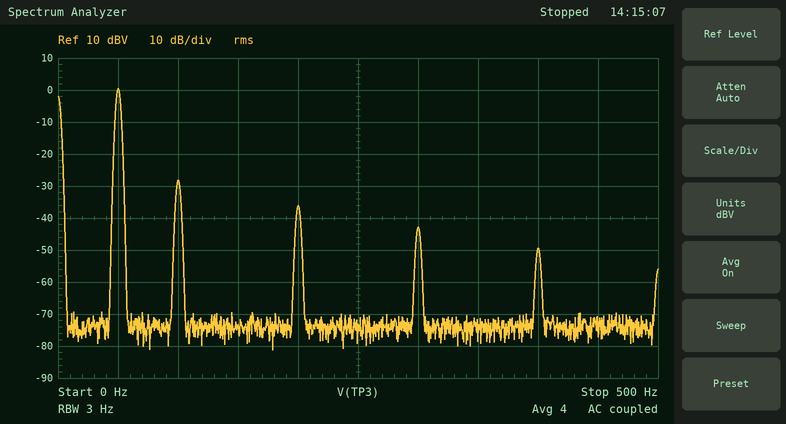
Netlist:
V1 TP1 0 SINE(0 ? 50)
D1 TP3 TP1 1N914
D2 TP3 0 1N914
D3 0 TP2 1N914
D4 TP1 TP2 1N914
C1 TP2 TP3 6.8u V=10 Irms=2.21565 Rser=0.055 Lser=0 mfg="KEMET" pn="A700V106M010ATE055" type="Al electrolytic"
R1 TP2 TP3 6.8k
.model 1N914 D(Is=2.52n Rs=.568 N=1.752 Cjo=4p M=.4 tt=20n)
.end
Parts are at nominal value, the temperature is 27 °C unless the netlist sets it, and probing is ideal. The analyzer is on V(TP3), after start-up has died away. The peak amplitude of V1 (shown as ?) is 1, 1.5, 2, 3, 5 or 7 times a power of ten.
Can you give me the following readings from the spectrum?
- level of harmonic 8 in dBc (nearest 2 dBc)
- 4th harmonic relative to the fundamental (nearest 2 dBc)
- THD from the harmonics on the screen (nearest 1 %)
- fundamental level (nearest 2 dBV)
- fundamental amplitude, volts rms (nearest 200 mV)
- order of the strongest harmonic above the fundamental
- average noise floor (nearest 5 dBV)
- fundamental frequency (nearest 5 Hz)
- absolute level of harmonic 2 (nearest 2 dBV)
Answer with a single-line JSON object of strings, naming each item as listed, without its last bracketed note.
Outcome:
{"level of harmonic 8 in dBc": "-50 dBc", "4th harmonic relative to the fundamental": "-36 dBc", "THD from the harmonics on the screen": "4 %", "fundamental level": "0 dBV", "fundamental amplitude, volts rms": "1.0 V", "order of the strongest harmonic above the fundamental": "2", "average noise floor": "-75 dBV", "fundamental frequency": "50 Hz", "absolute level of harmonic 2": "-28 dBV"}
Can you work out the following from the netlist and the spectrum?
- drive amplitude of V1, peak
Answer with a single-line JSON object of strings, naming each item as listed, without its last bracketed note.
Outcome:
{"drive amplitude of V1, peak": "3 V"}
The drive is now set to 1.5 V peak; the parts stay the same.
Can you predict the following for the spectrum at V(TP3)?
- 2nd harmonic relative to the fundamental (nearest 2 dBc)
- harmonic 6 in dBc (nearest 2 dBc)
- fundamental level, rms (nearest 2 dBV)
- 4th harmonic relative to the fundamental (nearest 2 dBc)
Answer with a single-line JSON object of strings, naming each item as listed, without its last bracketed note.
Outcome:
{"2nd harmonic relative to the fundamental": "-36 dBc", "harmonic 6 in dBc": "-54 dBc", "fundamental level, rms": "-6 dBV", "4th harmonic relative to the fundamental": "-44 dBc"}
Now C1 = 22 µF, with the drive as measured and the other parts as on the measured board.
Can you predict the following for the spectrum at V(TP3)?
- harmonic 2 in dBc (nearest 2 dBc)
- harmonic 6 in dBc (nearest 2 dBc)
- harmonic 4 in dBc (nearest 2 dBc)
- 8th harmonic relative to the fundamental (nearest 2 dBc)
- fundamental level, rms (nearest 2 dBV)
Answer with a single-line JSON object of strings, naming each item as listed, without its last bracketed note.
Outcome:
{"harmonic 2 in dBc": "-38 dBc", "harmonic 6 in dBc": "-52 dBc", "harmonic 4 in dBc": "-46 dBc", "8th harmonic relative to the fundamental": "-58 dBc", "fundamental level, rms": "0 dBV"}
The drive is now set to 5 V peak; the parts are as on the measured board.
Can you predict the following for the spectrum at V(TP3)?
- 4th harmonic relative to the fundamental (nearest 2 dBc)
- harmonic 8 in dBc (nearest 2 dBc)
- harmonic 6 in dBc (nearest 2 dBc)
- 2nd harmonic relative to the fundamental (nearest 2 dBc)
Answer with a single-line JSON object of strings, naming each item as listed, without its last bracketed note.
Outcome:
{"4th harmonic relative to the fundamental": "-34 dBc", "harmonic 8 in dBc": "-46 dBc", "harmonic 6 in dBc": "-40 dBc", "2nd harmonic relative to the fundamental": "-26 dBc"}
